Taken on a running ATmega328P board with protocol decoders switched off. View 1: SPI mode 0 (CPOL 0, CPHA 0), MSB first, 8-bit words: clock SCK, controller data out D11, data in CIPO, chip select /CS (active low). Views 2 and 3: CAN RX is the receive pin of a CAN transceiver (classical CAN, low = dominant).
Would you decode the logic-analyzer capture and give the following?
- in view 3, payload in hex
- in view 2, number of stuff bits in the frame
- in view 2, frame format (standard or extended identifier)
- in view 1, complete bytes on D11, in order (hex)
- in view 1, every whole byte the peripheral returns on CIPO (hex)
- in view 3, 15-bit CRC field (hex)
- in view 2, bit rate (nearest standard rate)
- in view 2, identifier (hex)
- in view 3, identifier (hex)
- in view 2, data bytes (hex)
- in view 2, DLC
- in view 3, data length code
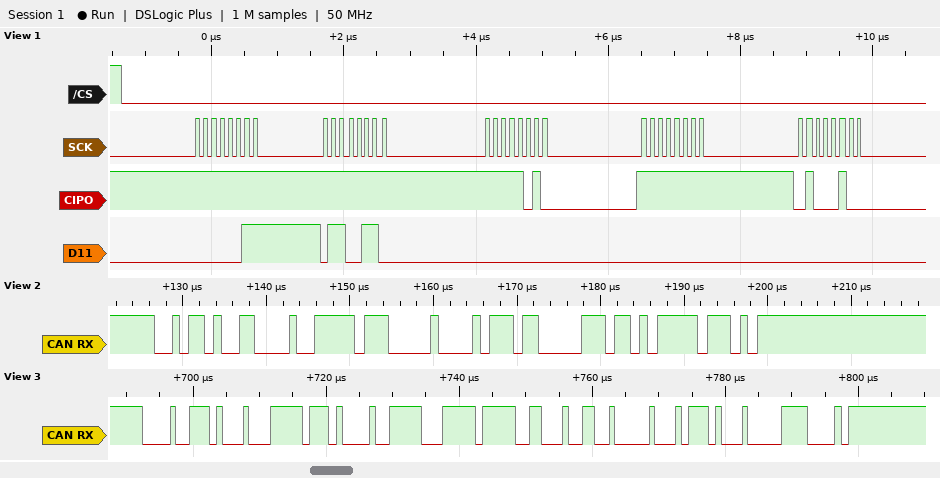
FF 42 7C FF D8 99 00 BA
4
standard
0x03 0x66 0x00 0x00 0x00
0xFF 0xFF 0xFA 0xFF 0x44
0x1070
1000 kbit/s
0x2D3
0x09D
FF 00 5D 83
4
8
